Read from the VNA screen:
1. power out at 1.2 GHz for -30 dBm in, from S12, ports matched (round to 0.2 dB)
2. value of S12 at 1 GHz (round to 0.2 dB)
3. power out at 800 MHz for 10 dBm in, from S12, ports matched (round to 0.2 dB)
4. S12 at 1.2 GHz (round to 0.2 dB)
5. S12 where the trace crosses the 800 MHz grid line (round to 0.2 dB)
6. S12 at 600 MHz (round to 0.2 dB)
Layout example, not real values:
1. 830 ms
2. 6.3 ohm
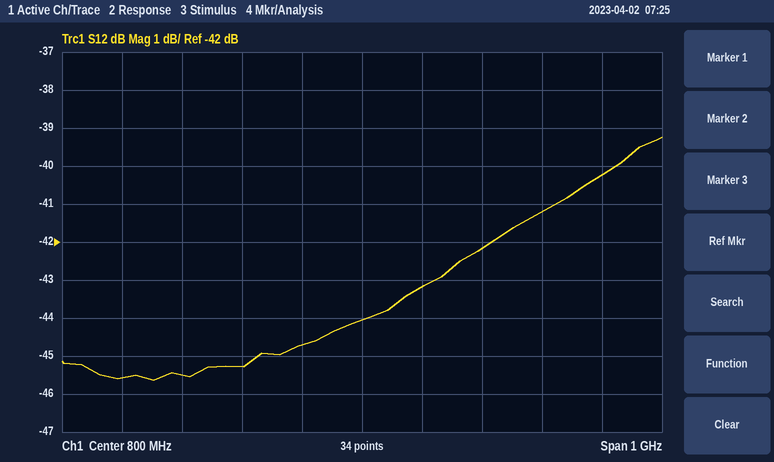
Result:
1. -70.2 dBm
2. -42.2 dB
3. -34.0 dBm
4. -40.2 dB
5. -44.0 dB
6. -45.2 dB
